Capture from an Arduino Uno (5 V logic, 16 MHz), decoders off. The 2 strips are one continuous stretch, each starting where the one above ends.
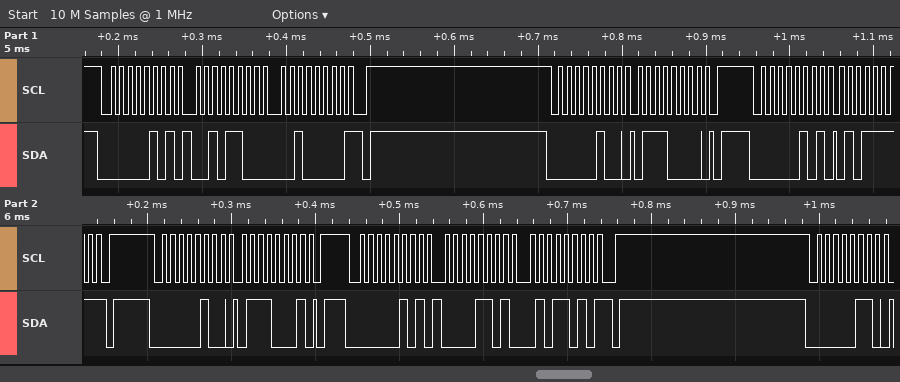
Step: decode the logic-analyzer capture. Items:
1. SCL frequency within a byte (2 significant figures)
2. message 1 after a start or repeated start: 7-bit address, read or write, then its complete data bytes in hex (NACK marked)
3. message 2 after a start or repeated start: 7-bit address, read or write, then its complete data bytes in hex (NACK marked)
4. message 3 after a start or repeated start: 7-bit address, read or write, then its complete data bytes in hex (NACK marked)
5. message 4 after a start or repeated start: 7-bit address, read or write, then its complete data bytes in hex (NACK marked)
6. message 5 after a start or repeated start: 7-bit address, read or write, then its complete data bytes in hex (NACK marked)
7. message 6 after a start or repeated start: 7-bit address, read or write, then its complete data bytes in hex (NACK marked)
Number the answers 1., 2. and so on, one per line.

1. 100 kHz
2. 0x02 read: 2C 20 NACK
3. 0x02 write: 70
4. 0x02 read: 5F NACK
5. 0x02 write: 71
6. 0x02 read: 0D 5A NACK
7. 0x03 write
